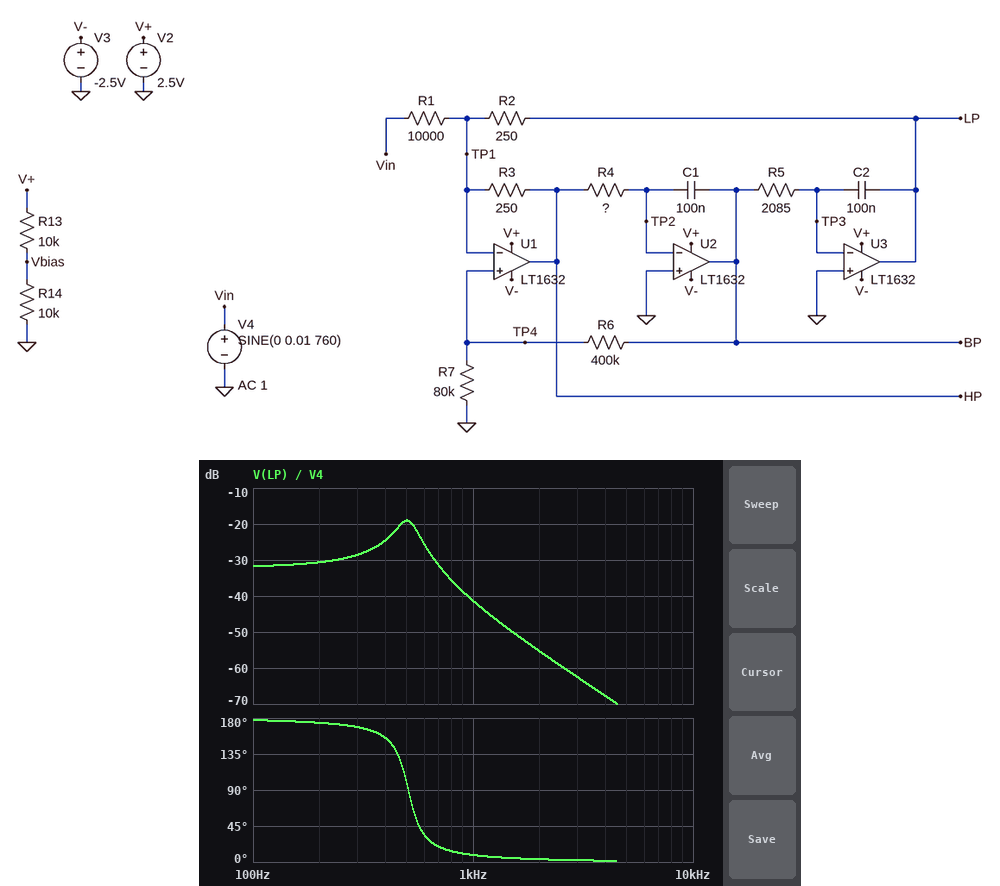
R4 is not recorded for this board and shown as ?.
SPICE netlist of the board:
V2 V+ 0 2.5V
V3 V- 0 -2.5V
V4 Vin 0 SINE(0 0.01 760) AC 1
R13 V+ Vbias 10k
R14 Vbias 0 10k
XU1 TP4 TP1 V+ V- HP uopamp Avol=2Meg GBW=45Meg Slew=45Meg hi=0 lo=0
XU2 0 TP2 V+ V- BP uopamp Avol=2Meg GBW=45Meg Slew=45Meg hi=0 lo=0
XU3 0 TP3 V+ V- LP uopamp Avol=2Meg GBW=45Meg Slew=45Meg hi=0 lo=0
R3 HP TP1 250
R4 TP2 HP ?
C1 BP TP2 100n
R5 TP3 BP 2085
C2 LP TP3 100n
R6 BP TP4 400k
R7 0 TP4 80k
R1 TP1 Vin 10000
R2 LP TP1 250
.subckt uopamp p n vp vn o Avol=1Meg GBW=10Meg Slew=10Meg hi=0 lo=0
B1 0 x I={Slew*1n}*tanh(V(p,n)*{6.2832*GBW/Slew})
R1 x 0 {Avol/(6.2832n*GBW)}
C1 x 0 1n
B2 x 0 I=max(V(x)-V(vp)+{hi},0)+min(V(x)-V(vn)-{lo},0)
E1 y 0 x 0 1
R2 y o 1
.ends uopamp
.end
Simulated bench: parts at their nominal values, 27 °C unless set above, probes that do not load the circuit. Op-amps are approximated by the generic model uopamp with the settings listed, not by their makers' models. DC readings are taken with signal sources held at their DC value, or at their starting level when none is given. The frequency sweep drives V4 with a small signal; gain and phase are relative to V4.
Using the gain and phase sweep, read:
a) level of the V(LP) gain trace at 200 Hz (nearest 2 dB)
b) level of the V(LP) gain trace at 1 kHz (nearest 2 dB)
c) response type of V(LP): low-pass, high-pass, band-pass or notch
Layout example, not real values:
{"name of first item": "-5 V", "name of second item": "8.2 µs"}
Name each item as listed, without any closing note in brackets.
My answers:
{"level of the V(LP) gain trace at 200 Hz": "-30 dB", "level of the V(LP) gain trace at 1 kHz": "-42 dB", "response type of V(LP): low-pass, high-pass, band-pass or notch": "low-pass"}
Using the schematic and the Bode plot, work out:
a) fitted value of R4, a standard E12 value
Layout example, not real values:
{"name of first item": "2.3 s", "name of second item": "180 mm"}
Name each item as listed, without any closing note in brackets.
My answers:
{"fitted value of R4, a standard E12 value": "4.7 kΩ"}
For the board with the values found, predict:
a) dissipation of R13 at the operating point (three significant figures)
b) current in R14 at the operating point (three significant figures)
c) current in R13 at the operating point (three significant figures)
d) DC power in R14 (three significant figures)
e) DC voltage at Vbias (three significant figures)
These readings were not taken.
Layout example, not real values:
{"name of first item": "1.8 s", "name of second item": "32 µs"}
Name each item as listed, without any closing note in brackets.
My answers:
{"dissipation of R13 at the operating point": "156 µW", "current in R14 at the operating point": "125 µA", "current in R13 at the operating point": "125 µA", "DC power in R14": "156 µW", "DC voltage at Vbias": "1.25 V"}
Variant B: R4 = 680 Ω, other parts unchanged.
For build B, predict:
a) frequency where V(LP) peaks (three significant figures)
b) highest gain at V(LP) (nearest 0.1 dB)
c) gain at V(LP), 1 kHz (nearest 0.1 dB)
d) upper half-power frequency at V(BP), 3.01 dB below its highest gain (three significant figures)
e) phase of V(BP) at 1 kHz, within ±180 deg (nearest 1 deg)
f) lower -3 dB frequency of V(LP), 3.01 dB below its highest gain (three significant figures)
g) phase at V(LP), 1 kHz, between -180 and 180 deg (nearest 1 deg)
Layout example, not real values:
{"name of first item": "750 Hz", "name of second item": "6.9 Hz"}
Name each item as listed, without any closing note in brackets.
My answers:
{"frequency where V(LP) peaks": "1.21 kHz", "highest gain at V(LP)": "-27.1 dB", "gain at V(LP), 1 kHz": "-27.9 dB", "upper half-power frequency at V(BP), 3.01 dB below its highest gain": "1.79 kHz", "phase of V(BP) at 1 kHz, within ±180 deg": "45 deg", "lower -3 dB frequency of V(LP), 3.01 dB below its highest gain": "683 Hz", "phase at V(LP), 1 kHz, between -180 and 180 deg": "135 deg"}
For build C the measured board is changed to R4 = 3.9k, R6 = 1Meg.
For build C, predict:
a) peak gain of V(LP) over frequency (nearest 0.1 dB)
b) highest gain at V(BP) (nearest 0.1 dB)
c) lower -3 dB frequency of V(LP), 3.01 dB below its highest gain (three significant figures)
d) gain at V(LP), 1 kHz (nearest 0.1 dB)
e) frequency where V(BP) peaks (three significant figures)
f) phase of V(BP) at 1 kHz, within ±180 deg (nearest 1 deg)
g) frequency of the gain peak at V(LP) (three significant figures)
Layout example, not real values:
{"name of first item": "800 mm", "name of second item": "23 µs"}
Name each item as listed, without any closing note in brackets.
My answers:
{"peak gain of V(LP) over frequency": "-12.8 dB", "highest gain at V(BP)": "-15.6 dB", "lower -3 dB frequency of V(LP), 3.01 dB below its highest gain": "525 Hz", "gain at V(LP), 1 kHz": "-39.0 dB", "frequency where V(BP) peaks": "558 Hz", "phase of V(BP) at 1 kHz, within ±180 deg": "-85 deg", "frequency of the gain peak at V(LP)": "556 Hz"}
